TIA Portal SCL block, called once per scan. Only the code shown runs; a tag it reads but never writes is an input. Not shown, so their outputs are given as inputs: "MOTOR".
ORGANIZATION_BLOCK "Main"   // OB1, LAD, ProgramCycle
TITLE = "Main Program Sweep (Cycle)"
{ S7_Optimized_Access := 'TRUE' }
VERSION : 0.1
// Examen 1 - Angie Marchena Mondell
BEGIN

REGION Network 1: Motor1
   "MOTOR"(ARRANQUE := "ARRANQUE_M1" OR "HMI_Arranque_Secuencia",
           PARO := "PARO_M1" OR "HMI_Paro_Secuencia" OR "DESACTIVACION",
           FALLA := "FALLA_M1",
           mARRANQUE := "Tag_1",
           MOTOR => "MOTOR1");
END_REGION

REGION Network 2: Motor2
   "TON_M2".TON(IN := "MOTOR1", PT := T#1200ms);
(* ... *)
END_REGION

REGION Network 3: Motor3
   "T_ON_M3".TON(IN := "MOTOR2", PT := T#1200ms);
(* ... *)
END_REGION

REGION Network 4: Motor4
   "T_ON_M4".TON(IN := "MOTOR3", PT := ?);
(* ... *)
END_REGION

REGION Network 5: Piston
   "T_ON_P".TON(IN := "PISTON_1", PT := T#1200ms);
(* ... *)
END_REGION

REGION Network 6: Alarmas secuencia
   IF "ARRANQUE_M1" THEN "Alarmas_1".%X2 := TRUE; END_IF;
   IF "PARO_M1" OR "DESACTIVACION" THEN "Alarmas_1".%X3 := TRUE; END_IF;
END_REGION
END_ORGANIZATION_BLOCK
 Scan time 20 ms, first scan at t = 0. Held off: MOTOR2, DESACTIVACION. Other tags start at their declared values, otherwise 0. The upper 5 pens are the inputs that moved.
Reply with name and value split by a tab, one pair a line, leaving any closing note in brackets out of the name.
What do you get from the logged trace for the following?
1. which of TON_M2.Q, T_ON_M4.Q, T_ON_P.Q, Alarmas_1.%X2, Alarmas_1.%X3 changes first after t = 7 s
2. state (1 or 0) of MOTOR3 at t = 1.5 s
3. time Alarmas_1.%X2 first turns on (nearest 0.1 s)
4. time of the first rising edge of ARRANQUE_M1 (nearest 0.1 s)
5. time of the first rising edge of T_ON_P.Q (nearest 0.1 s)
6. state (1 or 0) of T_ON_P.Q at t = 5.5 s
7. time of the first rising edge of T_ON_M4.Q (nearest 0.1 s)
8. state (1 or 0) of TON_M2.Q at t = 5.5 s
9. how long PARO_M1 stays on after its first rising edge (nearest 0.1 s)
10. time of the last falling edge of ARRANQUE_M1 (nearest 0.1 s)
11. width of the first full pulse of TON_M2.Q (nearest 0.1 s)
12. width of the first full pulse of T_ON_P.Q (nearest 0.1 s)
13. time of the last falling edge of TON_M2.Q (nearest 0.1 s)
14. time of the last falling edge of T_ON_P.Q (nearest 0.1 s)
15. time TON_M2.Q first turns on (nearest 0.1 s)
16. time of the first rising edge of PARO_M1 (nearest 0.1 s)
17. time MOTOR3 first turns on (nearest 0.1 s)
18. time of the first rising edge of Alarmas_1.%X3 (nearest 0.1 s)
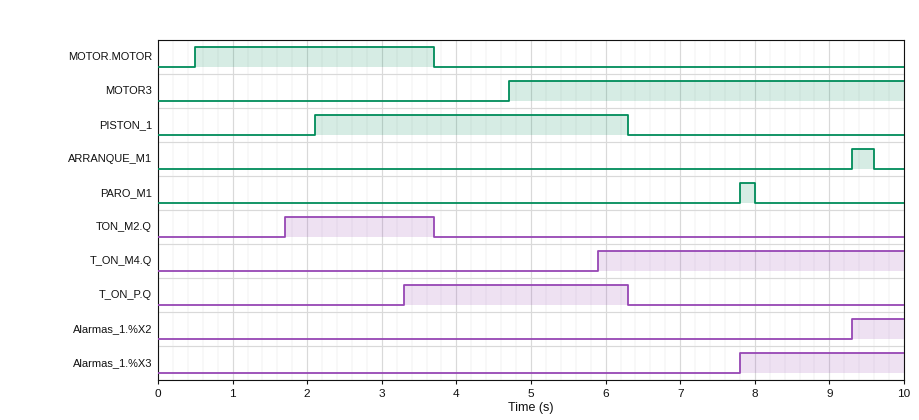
which of TON_M2.Q, T_ON_M4.Q, T_ON_P.Q, Alarmas_1.%X2, Alarmas_1.%X3 changes first after t = 7 s	Alarmas_1.%X3
state (1 or 0) of MOTOR3 at t = 1.5 s	0
time Alarmas_1.%X2 first turns on	9.3 s
time of the first rising edge of ARRANQUE_M1	9.3 s
time of the first rising edge of T_ON_P.Q	3.3 s
state (1 or 0) of T_ON_P.Q at t = 5.5 s	1
time of the first rising edge of T_ON_M4.Q	5.9 s
state (1 or 0) of TON_M2.Q at t = 5.5 s	0
how long PARO_M1 stays on after its first rising edge	0.2 s
time of the last falling edge of ARRANQUE_M1	9.6 s
width of the first full pulse of TON_M2.Q	2.0 s
width of the first full pulse of T_ON_P.Q	3.0 s
time of the last falling edge of TON_M2.Q	3.7 s
time of the last falling edge of T_ON_P.Q	6.3 s
time TON_M2.Q first turns on	1.7 s
time of the first rising edge of PARO_M1	7.8 s
time MOTOR3 first turns on	4.7 s
time of the first rising edge of Alarmas_1.%X3	7.8 s
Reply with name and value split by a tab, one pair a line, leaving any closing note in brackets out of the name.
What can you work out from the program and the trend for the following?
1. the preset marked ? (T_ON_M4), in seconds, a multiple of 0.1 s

the preset marked ? (T_ON_M4), in seconds, a multiple of 0.1 s	1.2 s
